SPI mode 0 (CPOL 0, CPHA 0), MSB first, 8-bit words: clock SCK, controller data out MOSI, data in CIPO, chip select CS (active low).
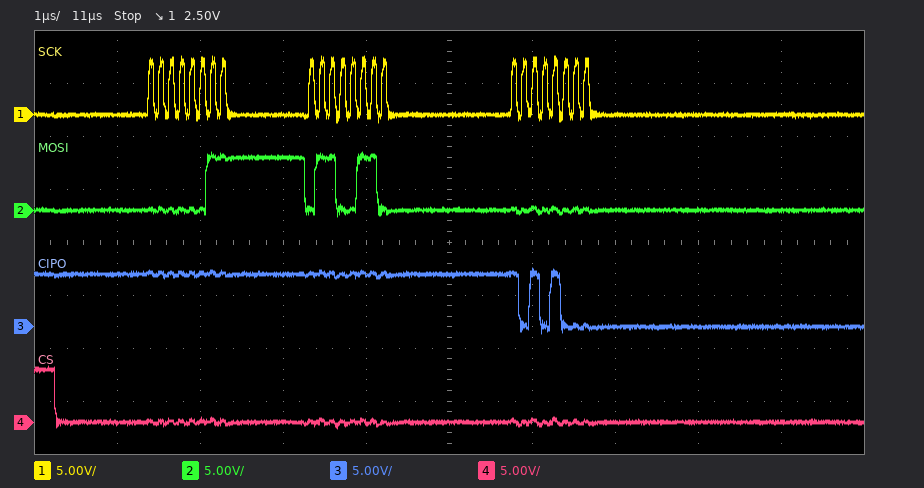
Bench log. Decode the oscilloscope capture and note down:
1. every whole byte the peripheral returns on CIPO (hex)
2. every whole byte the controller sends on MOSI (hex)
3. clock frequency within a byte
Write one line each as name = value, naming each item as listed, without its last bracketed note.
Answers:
every whole byte the peripheral returns on CIPO = FF FF A8
every whole byte the controller sends on MOSI = 03 66 00
clock frequency within a byte = 8 MHz
